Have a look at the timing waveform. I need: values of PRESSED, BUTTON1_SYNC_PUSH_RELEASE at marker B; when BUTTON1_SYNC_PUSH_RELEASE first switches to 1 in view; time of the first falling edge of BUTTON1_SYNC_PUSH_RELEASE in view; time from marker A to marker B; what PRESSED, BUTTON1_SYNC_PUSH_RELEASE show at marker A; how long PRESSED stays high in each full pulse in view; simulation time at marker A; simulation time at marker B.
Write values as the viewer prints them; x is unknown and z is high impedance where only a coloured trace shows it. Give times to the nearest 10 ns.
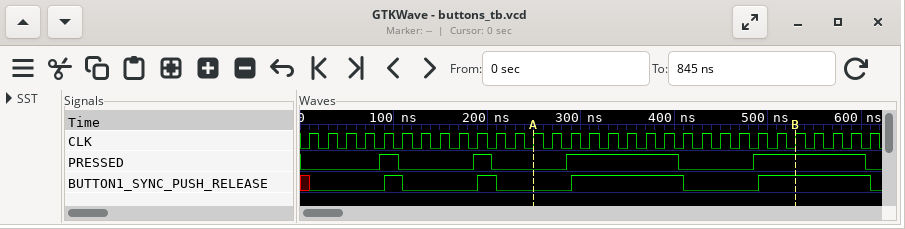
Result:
PRESSED=1, BUTTON1_SYNC_PUSH_RELEASE=1
90 ns
110 ns
280 ns
PRESSED=0, BUTTON1_SYNC_PUSH_RELEASE=0
20 ns, 20 ns, 120 ns, 120 ns
250 ns
530 ns
